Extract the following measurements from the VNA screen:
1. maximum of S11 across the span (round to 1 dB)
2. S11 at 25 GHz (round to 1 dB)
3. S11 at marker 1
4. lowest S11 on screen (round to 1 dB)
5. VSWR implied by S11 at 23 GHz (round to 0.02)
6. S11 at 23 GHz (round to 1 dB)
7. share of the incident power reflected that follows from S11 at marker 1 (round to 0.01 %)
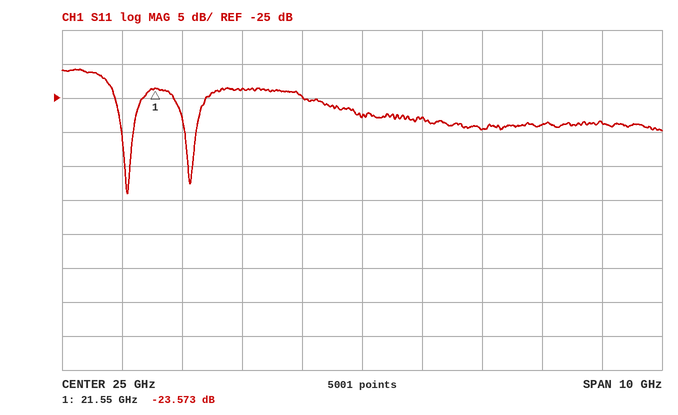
-21 dB
-28 dB
-23.573 dB
-39 dB
1.14
-24 dB
0.44 %
